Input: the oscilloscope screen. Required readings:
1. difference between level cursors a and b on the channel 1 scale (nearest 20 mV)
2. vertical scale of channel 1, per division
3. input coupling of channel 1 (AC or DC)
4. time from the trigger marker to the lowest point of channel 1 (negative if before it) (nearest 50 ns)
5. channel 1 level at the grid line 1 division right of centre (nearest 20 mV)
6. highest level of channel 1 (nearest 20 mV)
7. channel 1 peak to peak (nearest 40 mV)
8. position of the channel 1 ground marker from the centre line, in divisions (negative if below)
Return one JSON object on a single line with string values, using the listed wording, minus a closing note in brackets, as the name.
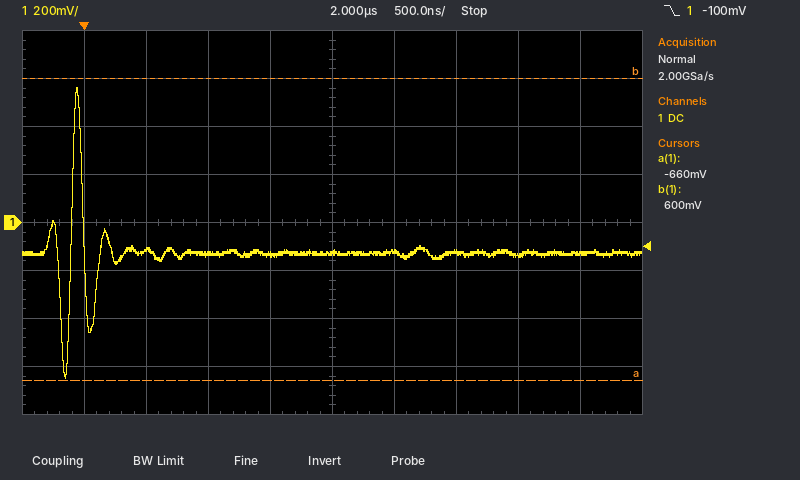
{"difference between level cursors a and b on the channel 1 scale": "1.26 V", "vertical scale of channel 1, per division": "200 mV", "input coupling of channel 1": "DC", "time from the trigger marker to the lowest point of channel 1 (negative if before it)": "-150 ns", "channel 1 level at the grid line 1 division right of centre": "-120 mV", "highest level of channel 1": "560 mV", "channel 1 peak to peak": "1.20 V", "position of the channel 1 ground marker from the centre line, in divisions": "0.0 div"}
